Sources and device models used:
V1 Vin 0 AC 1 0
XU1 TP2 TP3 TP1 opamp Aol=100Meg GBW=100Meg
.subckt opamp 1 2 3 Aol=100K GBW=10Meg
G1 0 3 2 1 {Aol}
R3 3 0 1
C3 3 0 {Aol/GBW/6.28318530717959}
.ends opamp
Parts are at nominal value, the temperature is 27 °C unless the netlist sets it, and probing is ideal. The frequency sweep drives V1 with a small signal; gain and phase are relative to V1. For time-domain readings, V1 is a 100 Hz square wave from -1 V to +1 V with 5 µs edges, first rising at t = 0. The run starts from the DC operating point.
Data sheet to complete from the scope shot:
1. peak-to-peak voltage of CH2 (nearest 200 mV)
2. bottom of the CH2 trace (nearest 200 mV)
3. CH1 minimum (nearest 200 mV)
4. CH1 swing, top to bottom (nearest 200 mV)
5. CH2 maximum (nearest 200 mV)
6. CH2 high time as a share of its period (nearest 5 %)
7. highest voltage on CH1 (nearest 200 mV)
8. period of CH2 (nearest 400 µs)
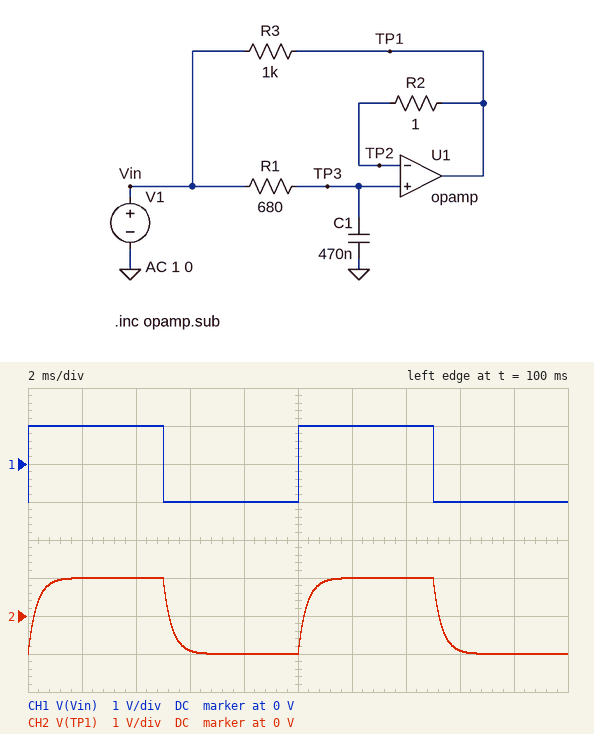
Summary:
2.0 V
-1.0 V
-1.0 V
2.0 V
1.0 V
50 %
1.0 V
10.0 ms
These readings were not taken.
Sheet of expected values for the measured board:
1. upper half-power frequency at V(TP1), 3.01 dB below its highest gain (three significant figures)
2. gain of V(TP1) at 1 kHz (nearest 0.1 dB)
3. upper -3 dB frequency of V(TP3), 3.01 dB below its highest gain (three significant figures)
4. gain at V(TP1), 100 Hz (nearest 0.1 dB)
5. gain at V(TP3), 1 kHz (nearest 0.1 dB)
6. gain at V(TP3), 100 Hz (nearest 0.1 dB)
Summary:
498 Hz
-7.0 dB
498 Hz
-0.2 dB
-7.0 dB
-0.2 dB
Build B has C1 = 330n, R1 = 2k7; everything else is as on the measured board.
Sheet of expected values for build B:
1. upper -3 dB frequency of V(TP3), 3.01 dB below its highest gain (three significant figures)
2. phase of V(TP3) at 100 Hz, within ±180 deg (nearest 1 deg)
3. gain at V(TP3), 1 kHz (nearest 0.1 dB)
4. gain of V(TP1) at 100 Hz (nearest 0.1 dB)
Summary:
179 Hz
-29 deg
-15.1 dB
-1.2 dB
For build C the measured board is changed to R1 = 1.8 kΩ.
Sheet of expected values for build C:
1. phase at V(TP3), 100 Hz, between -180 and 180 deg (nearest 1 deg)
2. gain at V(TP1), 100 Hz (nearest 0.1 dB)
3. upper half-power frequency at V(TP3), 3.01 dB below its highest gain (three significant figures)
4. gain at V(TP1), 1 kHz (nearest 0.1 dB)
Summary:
-28 deg
-1.1 dB
188 Hz
-14.7 dB
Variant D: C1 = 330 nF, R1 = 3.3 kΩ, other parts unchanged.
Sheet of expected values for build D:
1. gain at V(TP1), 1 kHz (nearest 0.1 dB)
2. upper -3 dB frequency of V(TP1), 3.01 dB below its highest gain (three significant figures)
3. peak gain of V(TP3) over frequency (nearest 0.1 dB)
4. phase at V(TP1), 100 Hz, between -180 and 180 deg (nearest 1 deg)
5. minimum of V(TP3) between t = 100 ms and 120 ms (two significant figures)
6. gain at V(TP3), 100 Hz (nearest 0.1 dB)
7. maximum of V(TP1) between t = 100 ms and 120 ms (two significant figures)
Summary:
-16.8 dB
146 Hz
0 dB
-34 deg
-980 mV
-1.7 dB
980 mV
